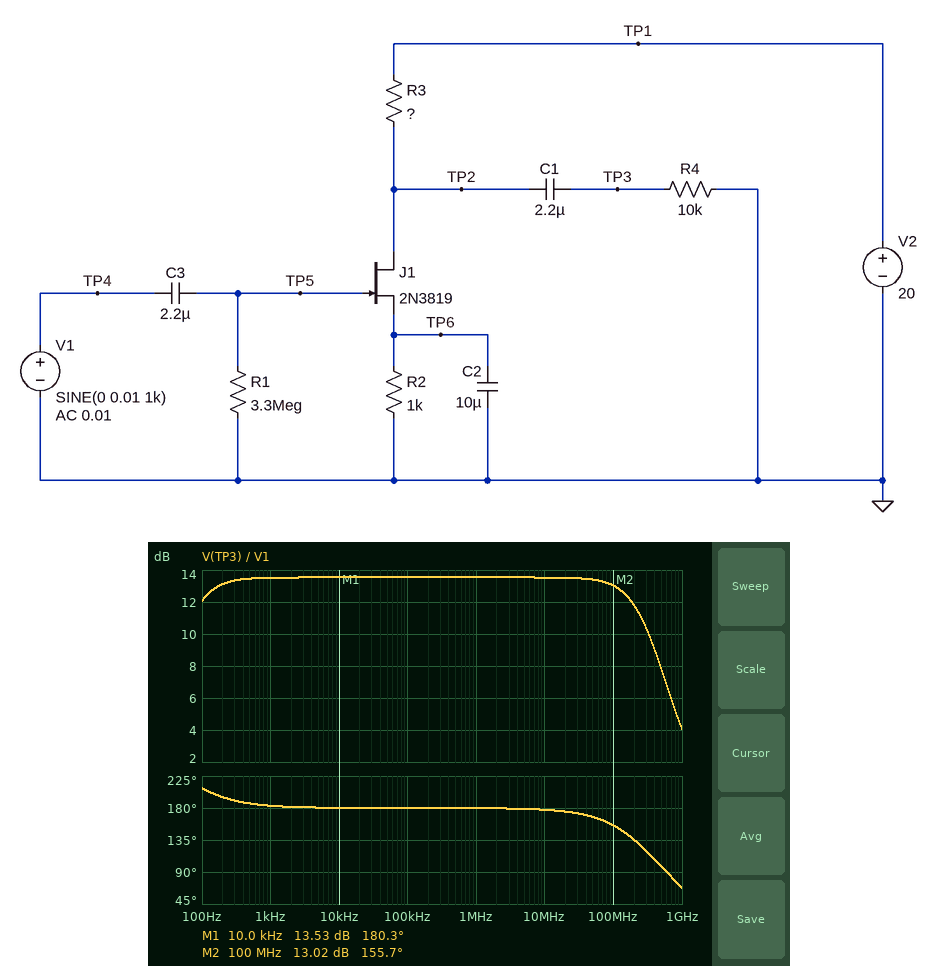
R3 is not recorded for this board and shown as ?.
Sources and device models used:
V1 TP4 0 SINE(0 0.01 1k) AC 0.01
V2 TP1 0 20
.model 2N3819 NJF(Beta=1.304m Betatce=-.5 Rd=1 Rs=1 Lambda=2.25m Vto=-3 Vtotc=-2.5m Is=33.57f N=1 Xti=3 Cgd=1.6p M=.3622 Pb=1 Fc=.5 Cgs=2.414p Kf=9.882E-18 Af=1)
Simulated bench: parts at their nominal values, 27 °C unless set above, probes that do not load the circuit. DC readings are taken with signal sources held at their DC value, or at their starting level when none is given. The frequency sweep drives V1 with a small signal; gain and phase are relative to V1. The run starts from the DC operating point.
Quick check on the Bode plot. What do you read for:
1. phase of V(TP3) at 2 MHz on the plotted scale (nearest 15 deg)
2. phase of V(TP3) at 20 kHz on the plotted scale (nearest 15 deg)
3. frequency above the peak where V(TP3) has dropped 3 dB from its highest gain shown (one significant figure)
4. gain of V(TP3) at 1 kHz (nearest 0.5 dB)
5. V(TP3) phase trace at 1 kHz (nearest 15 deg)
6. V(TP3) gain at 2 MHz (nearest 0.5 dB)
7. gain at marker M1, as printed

180 deg
180 deg
300 MHz
13.5 dB
180 deg
13.5 dB
13.53 dB
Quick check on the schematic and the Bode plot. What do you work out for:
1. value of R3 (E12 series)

1.8 kΩ
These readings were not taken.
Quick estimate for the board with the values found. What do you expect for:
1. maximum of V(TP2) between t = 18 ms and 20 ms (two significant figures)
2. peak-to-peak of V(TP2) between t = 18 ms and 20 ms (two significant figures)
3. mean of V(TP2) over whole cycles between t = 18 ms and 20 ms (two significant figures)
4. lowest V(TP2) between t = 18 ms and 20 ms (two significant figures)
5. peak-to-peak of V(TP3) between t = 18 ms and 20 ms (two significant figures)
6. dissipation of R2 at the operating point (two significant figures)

17 V
95 mV
17 V
17 V
95 mV
3.4 mW
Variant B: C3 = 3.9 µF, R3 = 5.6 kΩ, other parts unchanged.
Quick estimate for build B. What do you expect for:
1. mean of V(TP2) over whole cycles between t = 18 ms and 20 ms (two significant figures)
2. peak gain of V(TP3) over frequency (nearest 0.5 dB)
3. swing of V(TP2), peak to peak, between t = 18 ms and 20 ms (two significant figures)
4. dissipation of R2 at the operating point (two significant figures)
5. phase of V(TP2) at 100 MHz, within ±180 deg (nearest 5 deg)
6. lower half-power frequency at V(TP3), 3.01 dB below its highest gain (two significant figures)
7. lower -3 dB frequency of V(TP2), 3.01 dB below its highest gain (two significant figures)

9.8 V
21.0 dB
220 mV
3.3 mW
125 deg
61 Hz
60 Hz
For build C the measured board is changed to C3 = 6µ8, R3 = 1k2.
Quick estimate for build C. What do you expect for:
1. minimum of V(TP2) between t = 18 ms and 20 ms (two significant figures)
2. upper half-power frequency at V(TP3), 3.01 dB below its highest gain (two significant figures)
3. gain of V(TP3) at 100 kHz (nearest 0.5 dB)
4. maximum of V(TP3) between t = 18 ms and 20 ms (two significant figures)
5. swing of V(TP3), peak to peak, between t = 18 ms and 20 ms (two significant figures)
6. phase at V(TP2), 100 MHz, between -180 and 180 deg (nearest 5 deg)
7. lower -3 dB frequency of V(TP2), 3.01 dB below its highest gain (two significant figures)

18 V
450 MHz
10.5 dB
33 mV
67 mV
160 deg
62 Hz
